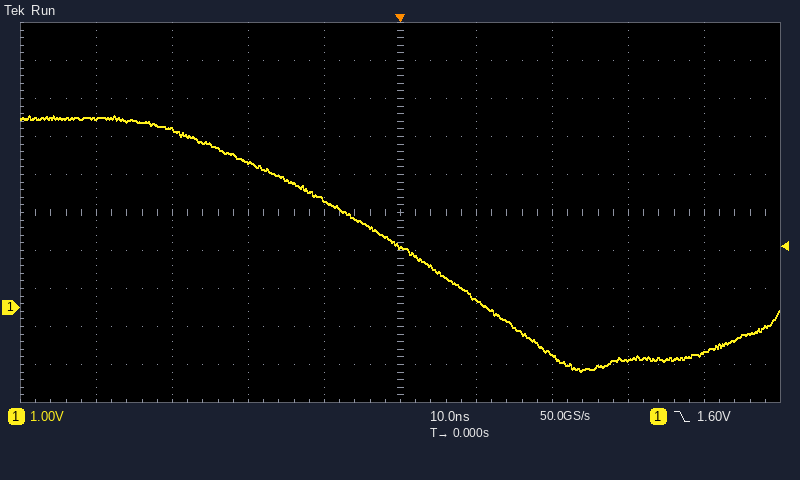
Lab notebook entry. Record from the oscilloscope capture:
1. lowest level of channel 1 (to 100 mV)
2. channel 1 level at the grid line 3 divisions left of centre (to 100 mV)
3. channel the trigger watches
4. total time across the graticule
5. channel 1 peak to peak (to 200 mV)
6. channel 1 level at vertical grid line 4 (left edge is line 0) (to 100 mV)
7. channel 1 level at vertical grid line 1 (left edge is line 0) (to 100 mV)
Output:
-1.7 V
4.7 V
channel 1
100 ns
6.8 V
2.8 V
5.0 V
